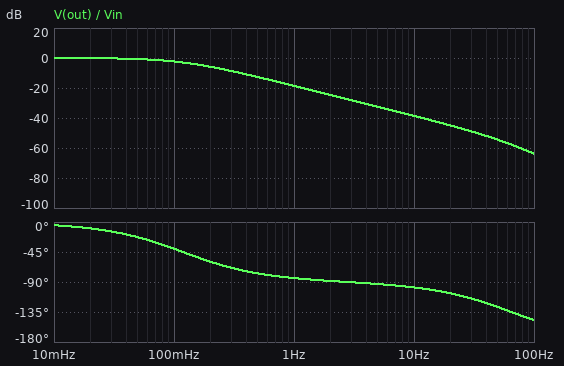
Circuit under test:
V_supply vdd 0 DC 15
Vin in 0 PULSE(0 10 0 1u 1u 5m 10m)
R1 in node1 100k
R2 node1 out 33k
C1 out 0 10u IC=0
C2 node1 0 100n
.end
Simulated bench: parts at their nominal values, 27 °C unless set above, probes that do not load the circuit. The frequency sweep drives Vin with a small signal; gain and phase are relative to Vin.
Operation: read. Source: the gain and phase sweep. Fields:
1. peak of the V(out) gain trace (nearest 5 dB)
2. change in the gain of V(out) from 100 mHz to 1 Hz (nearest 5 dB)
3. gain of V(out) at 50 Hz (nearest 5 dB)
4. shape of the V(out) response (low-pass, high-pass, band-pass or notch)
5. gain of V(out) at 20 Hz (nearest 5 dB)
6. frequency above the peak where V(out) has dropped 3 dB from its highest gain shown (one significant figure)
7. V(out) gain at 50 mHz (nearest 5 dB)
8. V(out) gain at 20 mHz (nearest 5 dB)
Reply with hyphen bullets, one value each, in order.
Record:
- 0 dB
- -15 dB
- -55 dB
- low-pass
- -45 dB
- 100 mHz
- 0 dB
- 0 dB
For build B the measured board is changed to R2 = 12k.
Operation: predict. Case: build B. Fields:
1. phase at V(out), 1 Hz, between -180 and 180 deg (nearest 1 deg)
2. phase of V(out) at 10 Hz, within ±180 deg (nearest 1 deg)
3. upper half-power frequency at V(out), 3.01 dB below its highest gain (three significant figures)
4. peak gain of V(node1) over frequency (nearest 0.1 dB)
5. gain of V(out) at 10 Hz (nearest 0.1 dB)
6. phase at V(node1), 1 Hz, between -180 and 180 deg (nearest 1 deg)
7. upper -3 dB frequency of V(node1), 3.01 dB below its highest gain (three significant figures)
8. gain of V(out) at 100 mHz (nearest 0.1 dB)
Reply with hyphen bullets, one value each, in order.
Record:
- -82 deg
- -93 deg
- 141 mHz
- 0 dB
- -37.0 dB
- -45 deg
- 143 mHz
- -1.8 dB
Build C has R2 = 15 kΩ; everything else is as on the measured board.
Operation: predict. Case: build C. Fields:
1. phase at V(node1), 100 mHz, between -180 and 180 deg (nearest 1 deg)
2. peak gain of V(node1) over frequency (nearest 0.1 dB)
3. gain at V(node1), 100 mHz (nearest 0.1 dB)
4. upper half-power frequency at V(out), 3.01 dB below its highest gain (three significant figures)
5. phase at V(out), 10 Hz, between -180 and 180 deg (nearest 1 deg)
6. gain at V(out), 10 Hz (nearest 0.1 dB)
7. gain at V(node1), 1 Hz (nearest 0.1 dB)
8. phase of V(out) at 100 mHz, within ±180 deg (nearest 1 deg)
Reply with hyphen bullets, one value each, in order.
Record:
- -31 deg
- 0 dB
- -1.8 dB
- 137 mHz
- -94 deg
- -37.3 dB
- -14.6 dB
- -36 deg
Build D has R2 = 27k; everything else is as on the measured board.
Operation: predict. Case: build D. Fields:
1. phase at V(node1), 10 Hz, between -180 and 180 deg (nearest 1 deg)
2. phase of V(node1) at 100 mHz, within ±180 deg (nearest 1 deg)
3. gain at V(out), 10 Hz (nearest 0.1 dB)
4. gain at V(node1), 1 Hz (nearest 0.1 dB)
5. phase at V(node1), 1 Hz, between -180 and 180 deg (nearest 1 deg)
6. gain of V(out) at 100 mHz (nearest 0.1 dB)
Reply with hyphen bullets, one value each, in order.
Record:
- -10 deg
- -29 deg
- -38.2 dB
- -12.3 dB
- -24 deg
- -2.2 dB
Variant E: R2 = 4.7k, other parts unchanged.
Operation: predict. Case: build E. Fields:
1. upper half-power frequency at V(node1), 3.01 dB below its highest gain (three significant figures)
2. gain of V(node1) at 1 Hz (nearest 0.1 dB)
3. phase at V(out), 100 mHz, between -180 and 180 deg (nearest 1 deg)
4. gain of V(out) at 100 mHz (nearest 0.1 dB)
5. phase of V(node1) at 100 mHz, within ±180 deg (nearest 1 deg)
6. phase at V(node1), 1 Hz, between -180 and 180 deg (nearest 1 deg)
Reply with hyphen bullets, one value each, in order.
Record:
- 151 mHz
- -16.2 dB
- -34 deg
- -1.6 dB
- -32 deg
- -65 deg
